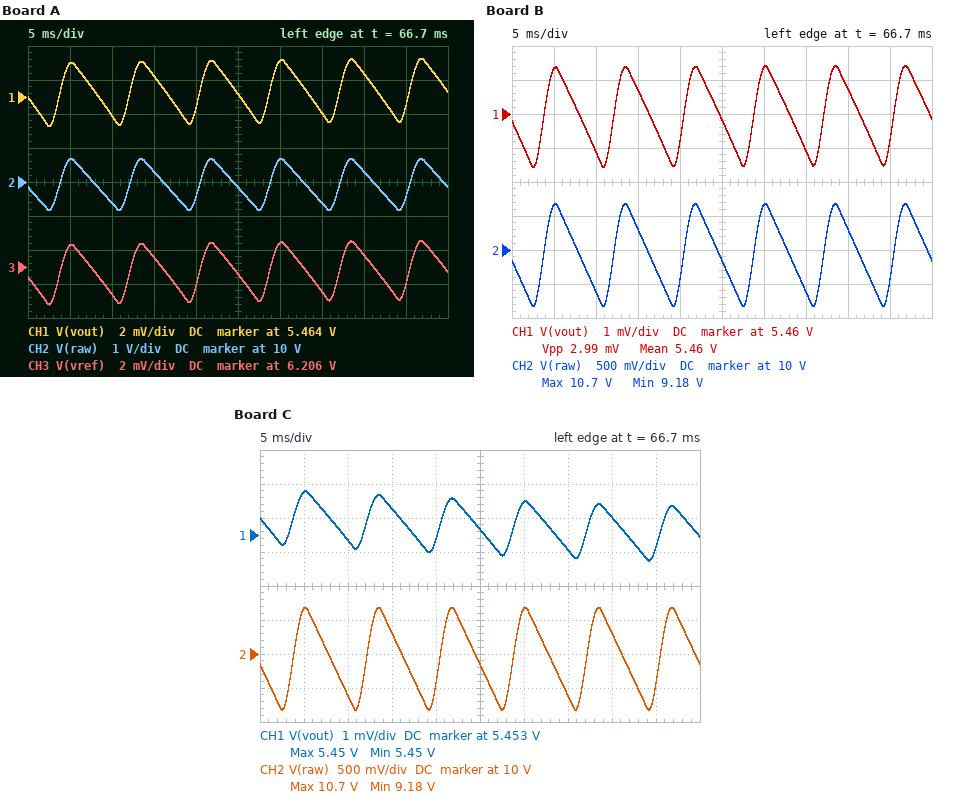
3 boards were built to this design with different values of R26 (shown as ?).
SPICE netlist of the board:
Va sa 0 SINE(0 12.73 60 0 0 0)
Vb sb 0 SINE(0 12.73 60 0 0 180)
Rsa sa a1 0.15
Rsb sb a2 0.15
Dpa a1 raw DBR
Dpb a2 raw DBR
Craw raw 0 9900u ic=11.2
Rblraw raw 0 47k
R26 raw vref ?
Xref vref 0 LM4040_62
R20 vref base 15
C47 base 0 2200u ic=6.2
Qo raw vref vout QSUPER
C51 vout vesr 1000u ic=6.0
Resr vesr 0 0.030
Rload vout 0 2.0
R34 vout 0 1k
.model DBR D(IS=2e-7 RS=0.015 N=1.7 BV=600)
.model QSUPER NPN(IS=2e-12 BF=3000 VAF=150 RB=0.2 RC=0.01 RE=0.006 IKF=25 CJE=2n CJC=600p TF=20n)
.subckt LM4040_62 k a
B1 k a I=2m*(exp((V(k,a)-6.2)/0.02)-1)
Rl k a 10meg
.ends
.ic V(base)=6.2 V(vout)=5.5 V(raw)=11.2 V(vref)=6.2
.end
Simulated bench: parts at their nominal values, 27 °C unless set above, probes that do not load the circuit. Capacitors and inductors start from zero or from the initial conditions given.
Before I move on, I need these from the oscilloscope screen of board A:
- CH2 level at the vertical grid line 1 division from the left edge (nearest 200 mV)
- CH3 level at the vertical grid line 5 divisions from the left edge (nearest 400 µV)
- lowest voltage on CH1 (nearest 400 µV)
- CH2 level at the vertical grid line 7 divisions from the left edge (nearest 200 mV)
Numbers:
10.6 V
6.2056 V
5.4624 V
9.4 V
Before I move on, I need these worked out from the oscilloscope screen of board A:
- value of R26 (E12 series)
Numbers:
2.2 kΩ
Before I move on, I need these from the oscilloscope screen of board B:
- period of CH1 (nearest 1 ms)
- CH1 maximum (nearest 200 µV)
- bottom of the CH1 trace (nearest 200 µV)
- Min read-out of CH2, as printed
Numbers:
8 ms
5.4614 V
5.4584 V
9.18 V
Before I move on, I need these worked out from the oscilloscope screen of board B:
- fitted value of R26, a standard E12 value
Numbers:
3.3 kΩ
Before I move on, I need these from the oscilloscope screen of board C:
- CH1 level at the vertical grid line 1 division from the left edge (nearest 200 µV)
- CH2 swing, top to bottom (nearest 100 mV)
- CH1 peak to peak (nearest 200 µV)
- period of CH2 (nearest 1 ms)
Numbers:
5.4542 V
1.5 V
2.0 mV
8 ms
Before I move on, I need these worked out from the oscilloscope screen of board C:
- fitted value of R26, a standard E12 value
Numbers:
8.2 kΩ
